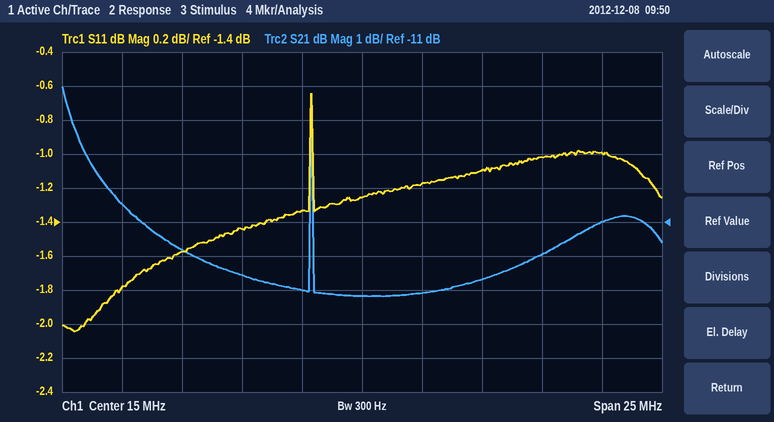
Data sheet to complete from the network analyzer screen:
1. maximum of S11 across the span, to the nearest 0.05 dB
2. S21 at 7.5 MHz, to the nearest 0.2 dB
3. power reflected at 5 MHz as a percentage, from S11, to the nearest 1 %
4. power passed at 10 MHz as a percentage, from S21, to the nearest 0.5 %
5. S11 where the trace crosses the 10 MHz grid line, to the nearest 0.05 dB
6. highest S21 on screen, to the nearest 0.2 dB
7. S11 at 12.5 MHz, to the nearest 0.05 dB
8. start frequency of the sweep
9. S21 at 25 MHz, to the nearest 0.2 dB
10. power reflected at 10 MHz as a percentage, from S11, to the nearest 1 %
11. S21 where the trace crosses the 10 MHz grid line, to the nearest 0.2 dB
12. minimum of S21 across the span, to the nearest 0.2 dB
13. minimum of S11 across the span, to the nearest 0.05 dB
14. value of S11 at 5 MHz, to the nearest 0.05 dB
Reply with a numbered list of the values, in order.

1. -0.65 dB
2. -11.8 dB
3. 66 %
4. 5.5 %
5. -1.45 dB
6. -7.0 dB
7. -1.35 dB
8. 2.5 MHz
9. -11.0 dB
10. 72 %
11. -12.6 dB
12. -13.2 dB
13. -2.05 dB
14. -1.80 dB
